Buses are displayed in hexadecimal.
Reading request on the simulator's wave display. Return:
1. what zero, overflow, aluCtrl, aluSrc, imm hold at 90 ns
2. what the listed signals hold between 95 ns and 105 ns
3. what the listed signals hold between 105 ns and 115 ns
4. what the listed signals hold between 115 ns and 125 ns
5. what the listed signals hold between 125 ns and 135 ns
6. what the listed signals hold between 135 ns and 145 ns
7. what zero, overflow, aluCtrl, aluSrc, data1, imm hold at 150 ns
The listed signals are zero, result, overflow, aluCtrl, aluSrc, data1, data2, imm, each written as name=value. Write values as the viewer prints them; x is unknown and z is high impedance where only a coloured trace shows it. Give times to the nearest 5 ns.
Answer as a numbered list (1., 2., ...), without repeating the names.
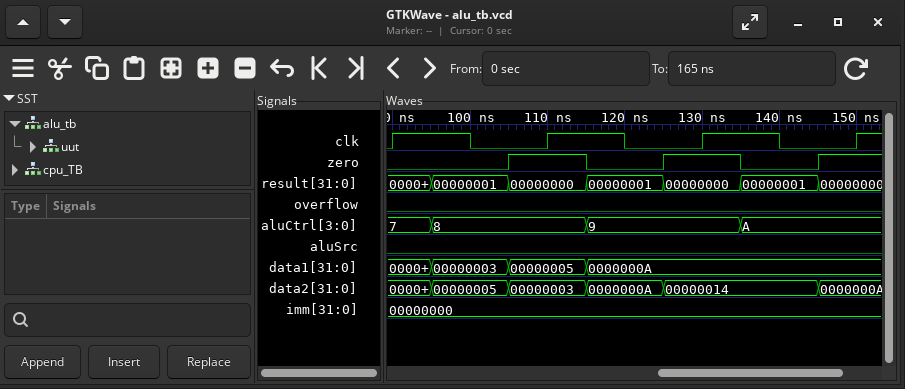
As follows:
1. zero=0, overflow=0, aluCtrl=7, aluSrc=0, imm=00000000
2. zero=0, result=00000001, overflow=0, aluCtrl=8, aluSrc=0, data1=00000003, data2=00000005, imm=00000000
3. zero=1, result=00000000, overflow=0, aluCtrl=8, aluSrc=0, data1=00000005, data2=00000003, imm=00000000
4. zero=0, result=00000001, overflow=0, aluCtrl=9, aluSrc=0, data1=0000000A, data2=0000000A, imm=00000000
5. zero=1, result=00000000, overflow=0, aluCtrl=9, aluSrc=0, data1=0000000A, data2=00000014, imm=00000000
6. zero=0, result=00000001, overflow=0, aluCtrl=A, aluSrc=0, data1=0000000A, data2=00000014, imm=00000000
7. zero=1, overflow=0, aluCtrl=A, aluSrc=0, data1=0000000A, imm=00000000
